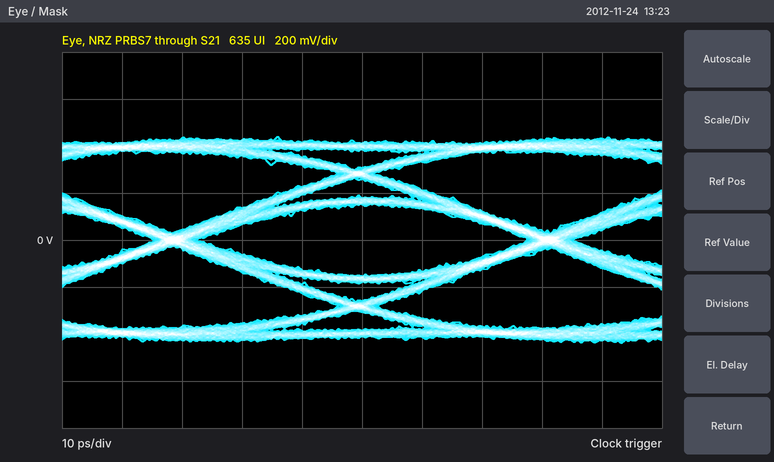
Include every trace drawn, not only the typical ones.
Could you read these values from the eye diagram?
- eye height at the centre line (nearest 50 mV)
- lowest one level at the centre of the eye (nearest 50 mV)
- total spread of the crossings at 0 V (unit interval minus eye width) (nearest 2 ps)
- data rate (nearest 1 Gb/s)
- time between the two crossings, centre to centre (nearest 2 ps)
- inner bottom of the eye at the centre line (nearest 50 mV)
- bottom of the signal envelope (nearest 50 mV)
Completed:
300 mV
150 mV
8 ps
16 Gb/s
62 ps
-150 mV
-450 mV
